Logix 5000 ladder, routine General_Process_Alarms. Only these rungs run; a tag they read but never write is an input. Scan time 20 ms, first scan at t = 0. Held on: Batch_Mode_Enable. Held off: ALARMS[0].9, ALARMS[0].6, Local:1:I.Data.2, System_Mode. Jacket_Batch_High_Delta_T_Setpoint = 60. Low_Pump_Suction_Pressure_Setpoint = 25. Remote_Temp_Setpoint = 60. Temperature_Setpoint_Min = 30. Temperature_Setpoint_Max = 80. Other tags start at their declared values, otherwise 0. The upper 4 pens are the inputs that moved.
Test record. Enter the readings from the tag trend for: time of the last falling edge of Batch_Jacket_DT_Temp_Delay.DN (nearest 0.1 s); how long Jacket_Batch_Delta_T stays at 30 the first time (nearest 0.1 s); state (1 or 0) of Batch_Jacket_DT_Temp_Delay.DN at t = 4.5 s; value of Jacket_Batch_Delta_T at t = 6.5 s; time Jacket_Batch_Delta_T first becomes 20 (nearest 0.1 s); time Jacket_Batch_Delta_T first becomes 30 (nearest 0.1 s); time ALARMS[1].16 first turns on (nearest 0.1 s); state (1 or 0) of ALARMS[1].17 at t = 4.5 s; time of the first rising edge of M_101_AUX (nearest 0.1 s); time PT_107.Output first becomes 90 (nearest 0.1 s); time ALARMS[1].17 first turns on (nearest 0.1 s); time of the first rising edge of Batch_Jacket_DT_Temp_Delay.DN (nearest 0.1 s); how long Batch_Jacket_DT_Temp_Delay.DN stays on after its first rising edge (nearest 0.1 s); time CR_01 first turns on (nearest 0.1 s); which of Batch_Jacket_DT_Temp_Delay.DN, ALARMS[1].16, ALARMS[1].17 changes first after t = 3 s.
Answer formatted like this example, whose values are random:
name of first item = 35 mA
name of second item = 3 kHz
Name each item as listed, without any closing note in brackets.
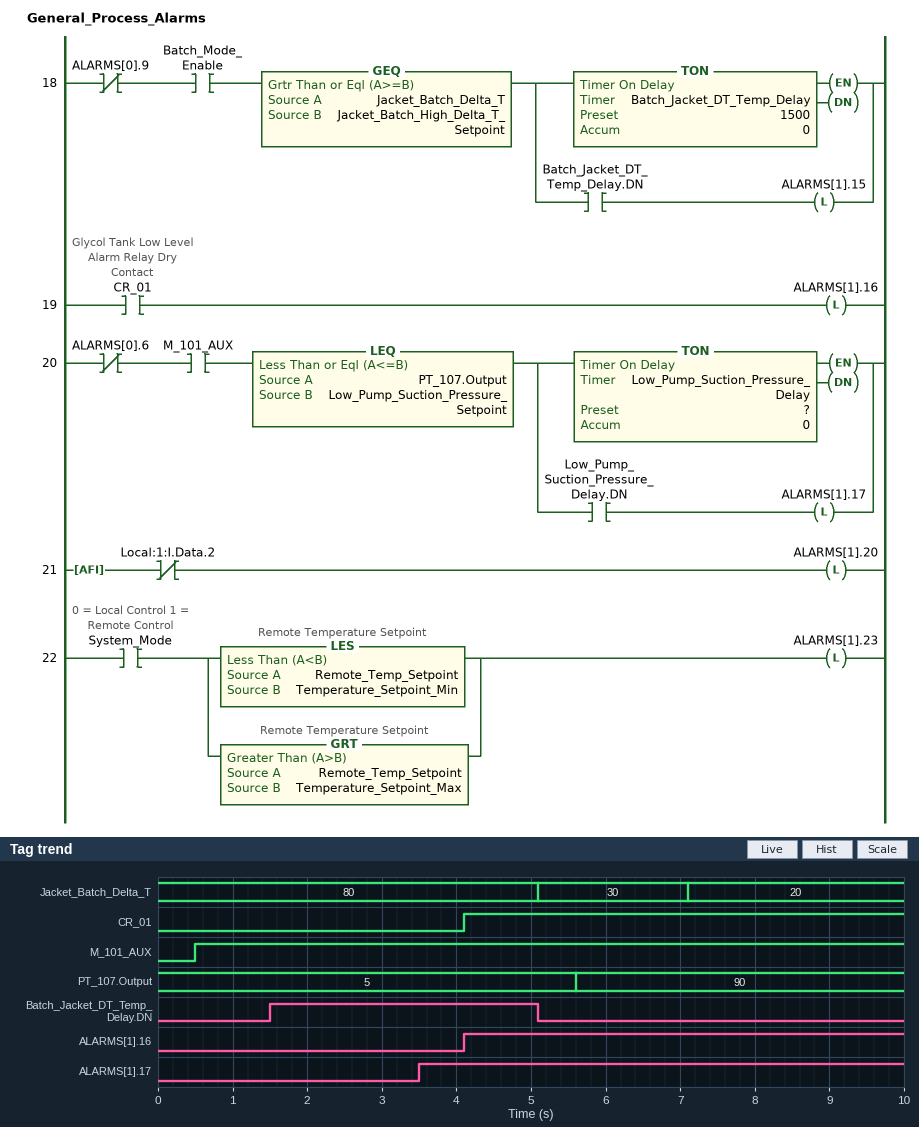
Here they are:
time of the last falling edge of Batch_Jacket_DT_Temp_Delay.DN = 5.1 s
how long Jacket_Batch_Delta_T stays at 30 the first time = 2.0 s
state (1 or 0) of Batch_Jacket_DT_Temp_Delay.DN at t = 4.5 s = 1
value of Jacket_Batch_Delta_T at t = 6.5 s = 30
time Jacket_Batch_Delta_T first becomes 20 = 7.1 s
time Jacket_Batch_Delta_T first becomes 30 = 5.1 s
time ALARMS[1].16 first turns on = 4.1 s
state (1 or 0) of ALARMS[1].17 at t = 4.5 s = 1
time of the first rising edge of M_101_AUX = 0.5 s
time PT_107.Output first becomes 90 = 5.6 s
time ALARMS[1].17 first turns on = 3.5 s
time of the first rising edge of Batch_Jacket_DT_Temp_Delay.DN = 1.5 s
how long Batch_Jacket_DT_Temp_Delay.DN stays on after its first rising edge = 3.6 s
time CR_01 first turns on = 4.1 s
which of Batch_Jacket_DT_Temp_Delay.DN, ALARMS[1].16, ALARMS[1].17 changes first after t = 3 s = ALARMS[1].17
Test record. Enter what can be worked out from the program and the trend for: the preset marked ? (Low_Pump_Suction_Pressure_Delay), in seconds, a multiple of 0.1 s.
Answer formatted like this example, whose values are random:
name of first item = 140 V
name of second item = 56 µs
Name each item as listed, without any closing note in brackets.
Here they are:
the preset marked ? (Low_Pump_Suction_Pressure_Delay), in seconds, a multiple of 0.1 s = 3.0 s
